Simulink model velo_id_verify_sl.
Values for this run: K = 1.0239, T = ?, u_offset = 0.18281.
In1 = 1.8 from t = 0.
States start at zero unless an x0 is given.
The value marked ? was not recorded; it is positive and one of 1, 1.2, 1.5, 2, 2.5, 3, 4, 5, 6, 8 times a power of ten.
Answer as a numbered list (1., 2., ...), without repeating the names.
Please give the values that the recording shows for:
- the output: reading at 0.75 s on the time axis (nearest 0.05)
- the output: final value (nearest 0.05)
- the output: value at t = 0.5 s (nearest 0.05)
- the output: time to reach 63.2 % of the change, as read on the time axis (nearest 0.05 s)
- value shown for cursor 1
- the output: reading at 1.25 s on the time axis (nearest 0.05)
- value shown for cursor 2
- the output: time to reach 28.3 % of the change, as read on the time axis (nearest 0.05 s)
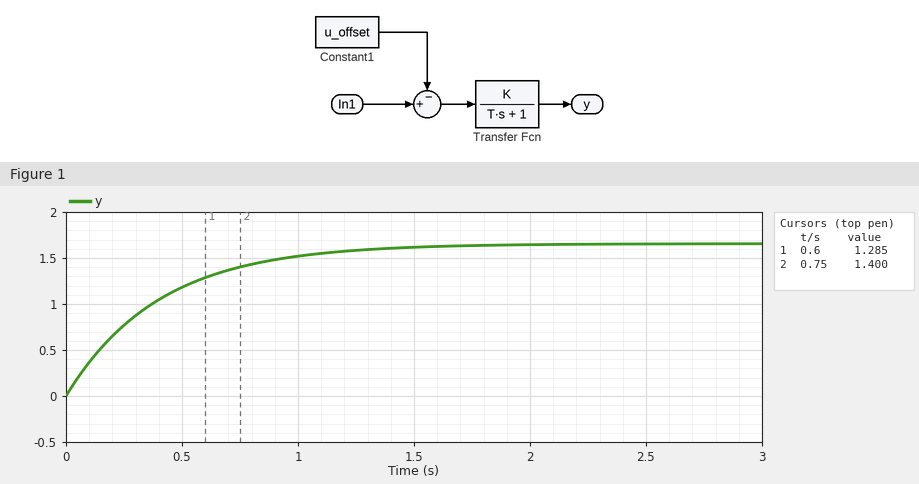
1. 1.40
2. 1.65
3. 1.20
4. 0.40 s
5. 1.285
6. 1.60
7. 1.400
8. 0.15 s
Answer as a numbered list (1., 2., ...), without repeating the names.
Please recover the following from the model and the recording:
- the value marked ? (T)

1. 0.4
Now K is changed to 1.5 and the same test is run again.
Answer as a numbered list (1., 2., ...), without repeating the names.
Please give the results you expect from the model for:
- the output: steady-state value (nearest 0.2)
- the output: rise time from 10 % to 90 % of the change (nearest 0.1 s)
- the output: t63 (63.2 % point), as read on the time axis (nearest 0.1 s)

1. 2.4
2. 0.9 s
3. 0.4 s
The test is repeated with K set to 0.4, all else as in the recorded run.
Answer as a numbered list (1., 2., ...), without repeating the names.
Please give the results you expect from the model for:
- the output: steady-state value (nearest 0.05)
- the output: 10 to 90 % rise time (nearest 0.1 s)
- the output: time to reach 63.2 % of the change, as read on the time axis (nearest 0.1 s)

1. 0.65
2. 0.9 s
3. 0.4 s
